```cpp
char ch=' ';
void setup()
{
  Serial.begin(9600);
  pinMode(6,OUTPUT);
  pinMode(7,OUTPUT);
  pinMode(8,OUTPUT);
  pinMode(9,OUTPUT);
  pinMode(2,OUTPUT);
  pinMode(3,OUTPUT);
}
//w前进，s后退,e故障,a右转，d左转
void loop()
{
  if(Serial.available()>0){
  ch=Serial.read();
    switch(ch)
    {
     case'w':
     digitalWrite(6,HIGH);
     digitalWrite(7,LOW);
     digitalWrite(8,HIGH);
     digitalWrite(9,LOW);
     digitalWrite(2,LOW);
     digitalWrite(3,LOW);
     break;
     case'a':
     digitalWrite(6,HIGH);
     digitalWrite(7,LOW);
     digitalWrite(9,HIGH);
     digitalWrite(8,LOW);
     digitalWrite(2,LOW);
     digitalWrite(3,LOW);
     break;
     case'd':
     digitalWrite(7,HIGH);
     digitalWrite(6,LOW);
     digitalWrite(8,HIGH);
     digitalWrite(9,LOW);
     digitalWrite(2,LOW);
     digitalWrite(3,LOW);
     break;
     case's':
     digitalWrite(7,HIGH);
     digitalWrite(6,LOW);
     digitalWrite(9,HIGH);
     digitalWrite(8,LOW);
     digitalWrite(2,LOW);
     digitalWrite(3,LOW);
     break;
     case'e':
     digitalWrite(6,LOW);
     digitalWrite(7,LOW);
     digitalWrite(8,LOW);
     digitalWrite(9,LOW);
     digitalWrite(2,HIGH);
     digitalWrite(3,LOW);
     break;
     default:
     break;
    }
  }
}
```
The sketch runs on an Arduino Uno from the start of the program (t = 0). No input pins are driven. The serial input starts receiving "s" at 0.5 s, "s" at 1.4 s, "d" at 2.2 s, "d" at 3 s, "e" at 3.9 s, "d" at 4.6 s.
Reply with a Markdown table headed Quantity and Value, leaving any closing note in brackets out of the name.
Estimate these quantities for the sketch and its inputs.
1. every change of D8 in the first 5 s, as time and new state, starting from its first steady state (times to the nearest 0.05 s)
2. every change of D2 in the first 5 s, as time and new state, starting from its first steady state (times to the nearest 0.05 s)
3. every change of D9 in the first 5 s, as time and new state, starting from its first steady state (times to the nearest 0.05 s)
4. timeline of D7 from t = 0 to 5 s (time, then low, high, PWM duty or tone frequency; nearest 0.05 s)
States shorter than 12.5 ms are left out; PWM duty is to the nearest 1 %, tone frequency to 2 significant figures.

| Quantity | Value |
|---|---|
| every change of D8 in the first 5 s, as time and new state, starting from its first steady state | 0 s low; 2.2 s high; 3.9 s low; 4.6 s high |
| every change of D2 in the first 5 s, as time and new state, starting from its first steady state | 0 s low; 3.9 s high; 4.6 s low |
| every change of D9 in the first 5 s, as time and new state, starting from its first steady state | 0 s low; 0.5 s high; 2.2 s low |
| timeline of D7 from t = 0 to 5 s | 0 s low; 0.5 s high; 3.9 s low; 4.6 s high |
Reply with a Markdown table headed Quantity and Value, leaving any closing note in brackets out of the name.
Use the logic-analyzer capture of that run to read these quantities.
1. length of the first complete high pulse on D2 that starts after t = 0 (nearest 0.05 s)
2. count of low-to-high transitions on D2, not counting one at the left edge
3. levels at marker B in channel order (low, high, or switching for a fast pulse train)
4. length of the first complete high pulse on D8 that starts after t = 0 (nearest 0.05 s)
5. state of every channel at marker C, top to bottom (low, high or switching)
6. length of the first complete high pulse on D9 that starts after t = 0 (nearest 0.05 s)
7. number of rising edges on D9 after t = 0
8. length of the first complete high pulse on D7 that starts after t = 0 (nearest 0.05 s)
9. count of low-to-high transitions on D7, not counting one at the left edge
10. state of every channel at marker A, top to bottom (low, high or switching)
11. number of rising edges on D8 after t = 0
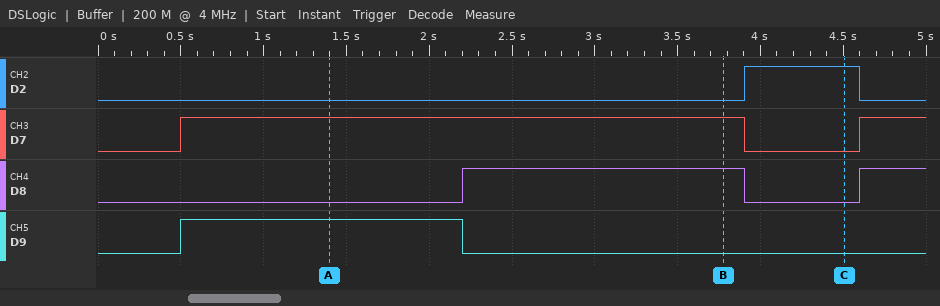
| Quantity | Value |
|---|---|
| length of the first complete high pulse on D2 that starts after t = 0 | 0.70 s |
| count of low-to-high transitions on D2, not counting one at the left edge | 1 |
| levels at marker B in channel order | D2 low, D7 high, D8 high, D9 low |
| length of the first complete high pulse on D8 that starts after t = 0 | 1.70 s |
| state of every channel at marker C, top to bottom | D2 high, D7 low, D8 low, D9 low |
| length of the first complete high pulse on D9 that starts after t = 0 | 1.70 s |
| number of rising edges on D9 after t = 0 | 1 |
| length of the first complete high pulse on D7 that starts after t = 0 | 3.40 s |
| count of low-to-high transitions on D7, not counting one at the left edge | 2 |
| state of every channel at marker A, top to bottom | D2 low, D7 high, D8 low, D9 high |
| number of rising edges on D8 after t = 0 | 2 |
